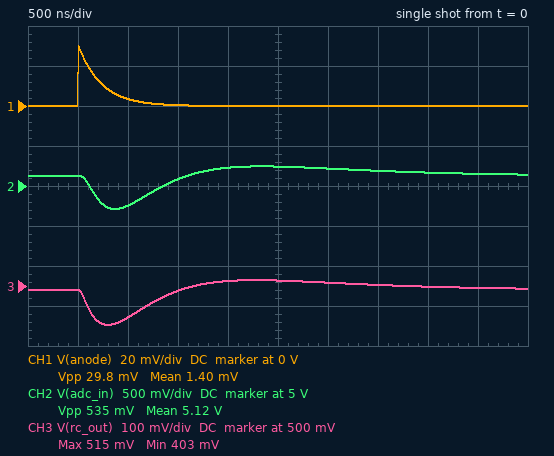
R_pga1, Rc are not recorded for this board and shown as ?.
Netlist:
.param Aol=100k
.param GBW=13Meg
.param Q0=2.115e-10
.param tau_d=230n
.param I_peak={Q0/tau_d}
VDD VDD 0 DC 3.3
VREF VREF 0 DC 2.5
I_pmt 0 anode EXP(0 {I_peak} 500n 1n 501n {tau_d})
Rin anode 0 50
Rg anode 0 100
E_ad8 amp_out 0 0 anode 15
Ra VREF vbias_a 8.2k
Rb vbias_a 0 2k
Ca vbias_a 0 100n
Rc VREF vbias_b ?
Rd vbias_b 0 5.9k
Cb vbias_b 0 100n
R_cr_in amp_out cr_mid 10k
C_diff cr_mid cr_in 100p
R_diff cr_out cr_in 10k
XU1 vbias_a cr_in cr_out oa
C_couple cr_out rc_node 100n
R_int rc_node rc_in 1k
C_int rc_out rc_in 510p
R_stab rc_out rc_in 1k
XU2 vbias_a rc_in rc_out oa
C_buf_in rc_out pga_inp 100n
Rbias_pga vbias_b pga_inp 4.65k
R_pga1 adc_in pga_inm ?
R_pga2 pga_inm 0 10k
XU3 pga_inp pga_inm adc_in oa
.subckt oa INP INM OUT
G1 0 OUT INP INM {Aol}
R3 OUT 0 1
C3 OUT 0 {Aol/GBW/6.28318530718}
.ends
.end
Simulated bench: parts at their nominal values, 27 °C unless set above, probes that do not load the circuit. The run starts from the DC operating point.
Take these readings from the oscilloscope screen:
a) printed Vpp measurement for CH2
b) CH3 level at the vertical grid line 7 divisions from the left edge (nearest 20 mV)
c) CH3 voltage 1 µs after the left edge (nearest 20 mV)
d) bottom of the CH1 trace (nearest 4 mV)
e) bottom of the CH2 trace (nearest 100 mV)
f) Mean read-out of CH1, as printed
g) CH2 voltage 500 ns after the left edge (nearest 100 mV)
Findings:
535 mV
500 mV
420 mV
0 V
4.7 V
1.40 mV
5.1 V
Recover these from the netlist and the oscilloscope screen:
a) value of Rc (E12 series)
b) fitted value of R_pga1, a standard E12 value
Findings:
8.2 kΩ
39 kΩ
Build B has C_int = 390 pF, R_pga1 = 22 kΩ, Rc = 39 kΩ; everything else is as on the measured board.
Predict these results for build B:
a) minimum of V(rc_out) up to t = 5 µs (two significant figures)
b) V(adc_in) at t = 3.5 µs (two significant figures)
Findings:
390 mV
1.1 V
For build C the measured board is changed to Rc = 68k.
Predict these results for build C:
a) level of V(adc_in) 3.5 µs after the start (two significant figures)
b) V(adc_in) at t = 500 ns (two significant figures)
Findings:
1.0 V
980 mV
